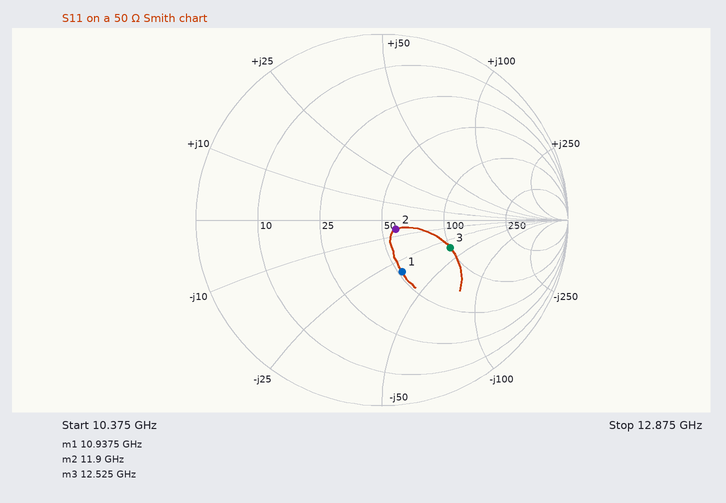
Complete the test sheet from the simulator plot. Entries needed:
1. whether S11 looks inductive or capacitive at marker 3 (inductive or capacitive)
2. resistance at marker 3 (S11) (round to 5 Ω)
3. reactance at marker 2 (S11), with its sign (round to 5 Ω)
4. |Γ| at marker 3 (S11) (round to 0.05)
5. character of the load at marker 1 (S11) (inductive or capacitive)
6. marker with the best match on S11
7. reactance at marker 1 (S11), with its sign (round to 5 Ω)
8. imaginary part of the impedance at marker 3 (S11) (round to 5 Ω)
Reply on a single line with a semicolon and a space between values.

capacitive; 100 Ω; -5 Ω; 0.40; capacitive; marker 2; -30 Ω; -35 Ω
